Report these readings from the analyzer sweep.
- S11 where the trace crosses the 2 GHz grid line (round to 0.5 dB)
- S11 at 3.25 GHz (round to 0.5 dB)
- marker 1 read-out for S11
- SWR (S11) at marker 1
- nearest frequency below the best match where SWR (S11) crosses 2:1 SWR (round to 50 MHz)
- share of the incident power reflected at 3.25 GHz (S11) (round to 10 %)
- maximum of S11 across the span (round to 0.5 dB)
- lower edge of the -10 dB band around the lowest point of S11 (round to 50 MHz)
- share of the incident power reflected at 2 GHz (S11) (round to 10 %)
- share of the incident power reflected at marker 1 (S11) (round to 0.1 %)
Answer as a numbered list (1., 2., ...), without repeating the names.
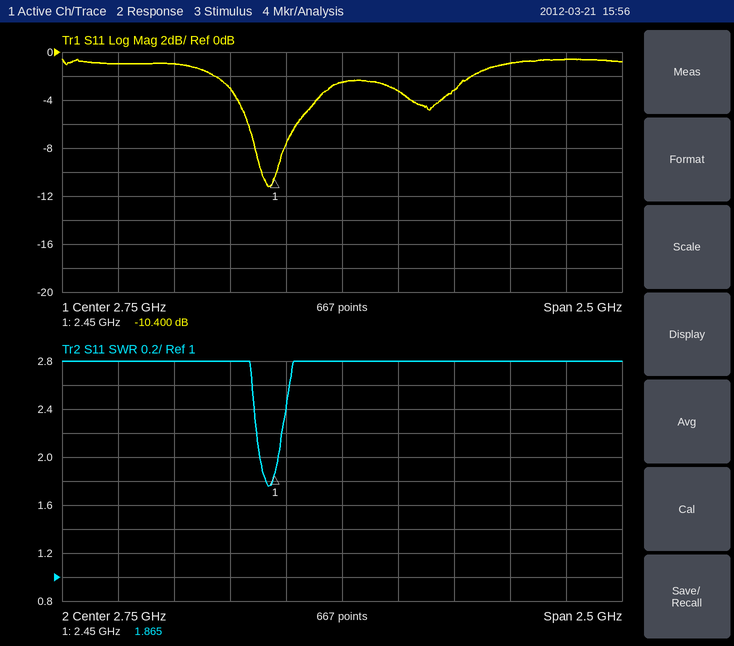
1. -1.0 dB
2. -3.0 dB
3. -10.400 dB
4. 1.865
5. 2.40 GHz
6. 50 %
7. -0.5 dB
8. 2.40 GHz
9. 80 %
10. 9.1 %
